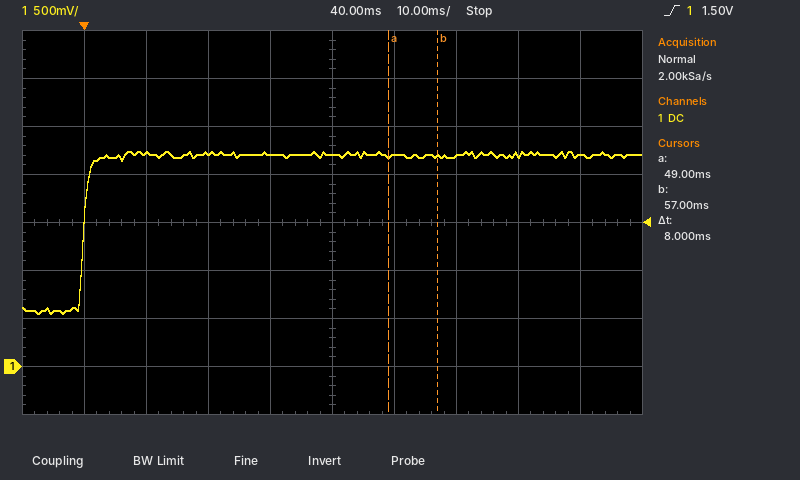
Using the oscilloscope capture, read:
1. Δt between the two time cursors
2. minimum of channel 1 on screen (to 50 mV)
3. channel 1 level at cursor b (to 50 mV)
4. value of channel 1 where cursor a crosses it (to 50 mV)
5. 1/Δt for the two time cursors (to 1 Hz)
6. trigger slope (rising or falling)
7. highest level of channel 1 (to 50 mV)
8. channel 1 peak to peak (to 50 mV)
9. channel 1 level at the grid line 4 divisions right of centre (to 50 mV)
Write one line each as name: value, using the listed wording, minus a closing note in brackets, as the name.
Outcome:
Δt between the two time cursors: 8 ms
minimum of channel 1 on screen: 550 mV
channel 1 level at cursor b: 2.20 V
value of channel 1 where cursor a crosses it: 2.20 V
1/Δt for the two time cursors: 125 Hz
trigger slope: rising
highest level of channel 1: 2.25 V
channel 1 peak to peak: 1.70 V
channel 1 level at the grid line 4 divisions right of centre: 2.20 V
